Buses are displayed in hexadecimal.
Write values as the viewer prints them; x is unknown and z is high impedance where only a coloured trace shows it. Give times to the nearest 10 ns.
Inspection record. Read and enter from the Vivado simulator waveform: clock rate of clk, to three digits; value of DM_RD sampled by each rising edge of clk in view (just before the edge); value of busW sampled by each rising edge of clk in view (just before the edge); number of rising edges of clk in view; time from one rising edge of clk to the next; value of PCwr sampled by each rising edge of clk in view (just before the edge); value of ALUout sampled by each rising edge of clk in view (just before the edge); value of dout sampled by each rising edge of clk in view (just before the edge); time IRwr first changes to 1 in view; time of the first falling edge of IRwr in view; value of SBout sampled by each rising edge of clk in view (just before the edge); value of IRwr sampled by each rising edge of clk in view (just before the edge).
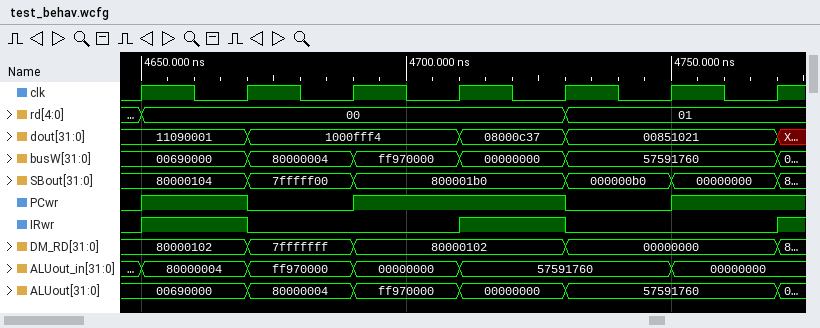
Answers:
50.0 MHz
80000102, 80000102, 7fffffff, 80000102, 80000102, 00000000, 00000000
00690000, 00690000, 80000004, ff970000, 00000000, 57591760, 57591760
7
20 ns
0 1 0 1 1 0 1
00690000, 00690000, 80000004, ff970000, 00000000, 57591760, 57591760
11090001, 11090001, 1000fff4, 1000fff4, 08000c37, 00851021, 00851021
4650 ns
4670 ns
80000104, 80000104, 7fffff00, 800001b0, 800001b0, 000000b0, 00000000
0 1 0 0 1 0 0
